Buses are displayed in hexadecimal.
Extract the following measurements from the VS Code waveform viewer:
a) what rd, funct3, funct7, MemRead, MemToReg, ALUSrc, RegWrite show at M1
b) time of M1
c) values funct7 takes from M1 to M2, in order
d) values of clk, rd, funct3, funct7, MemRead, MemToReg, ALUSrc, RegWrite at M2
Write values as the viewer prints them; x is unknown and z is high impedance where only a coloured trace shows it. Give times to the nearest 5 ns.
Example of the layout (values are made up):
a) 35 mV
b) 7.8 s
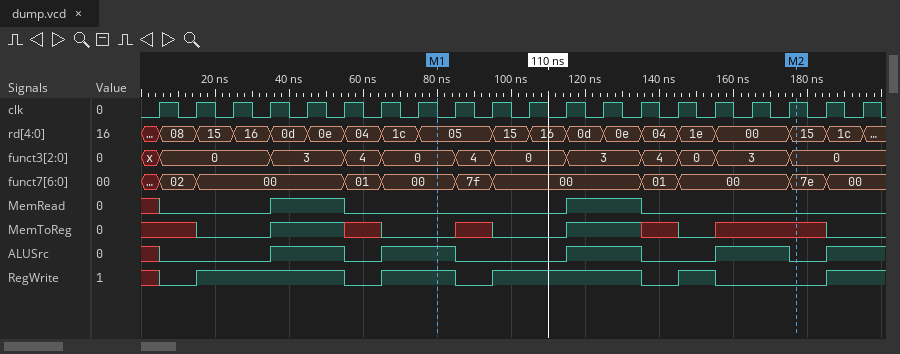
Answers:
a) rd=05, funct3=0, funct7=00, MemRead=0, MemToReg=0, ALUSrc=1, RegWrite=1
b) 80 ns
c) 00, 7f, 00, 01, 00, 7e
d) clk=1, rd=15, funct3=0, funct7=7e, MemRead=0, MemToReg=x, ALUSrc=0, RegWrite=0
